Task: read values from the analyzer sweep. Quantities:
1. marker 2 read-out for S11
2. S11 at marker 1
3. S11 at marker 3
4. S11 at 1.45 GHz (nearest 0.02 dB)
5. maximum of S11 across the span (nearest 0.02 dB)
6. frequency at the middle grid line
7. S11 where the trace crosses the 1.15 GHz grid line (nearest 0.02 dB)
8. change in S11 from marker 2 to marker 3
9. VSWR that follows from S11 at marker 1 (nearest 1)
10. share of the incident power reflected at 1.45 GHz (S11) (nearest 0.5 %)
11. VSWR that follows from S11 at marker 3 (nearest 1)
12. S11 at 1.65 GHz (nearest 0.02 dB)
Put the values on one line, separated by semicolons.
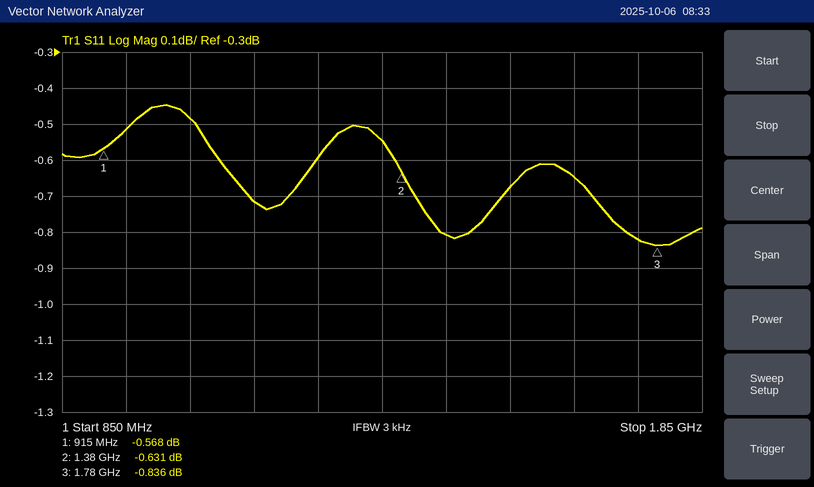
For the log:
-0.631 dB; -0.568 dB; -0.836 dB; -0.80 dB; -0.44 dB; 1.35 GHz; -0.72 dB; -0.205 dB; 31; 83.0 %; 21; -0.64 dB
